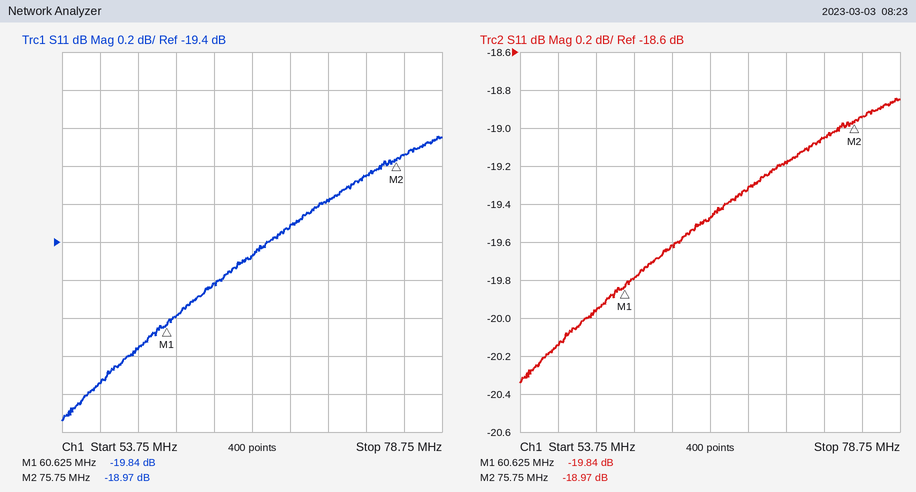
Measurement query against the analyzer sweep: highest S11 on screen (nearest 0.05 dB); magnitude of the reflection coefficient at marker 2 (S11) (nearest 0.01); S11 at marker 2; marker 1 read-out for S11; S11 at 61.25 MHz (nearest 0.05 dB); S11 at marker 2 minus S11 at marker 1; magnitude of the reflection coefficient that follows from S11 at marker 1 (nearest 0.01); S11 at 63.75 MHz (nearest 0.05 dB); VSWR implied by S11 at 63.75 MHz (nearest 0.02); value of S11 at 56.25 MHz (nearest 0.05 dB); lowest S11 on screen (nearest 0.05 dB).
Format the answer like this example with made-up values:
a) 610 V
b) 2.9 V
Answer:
a) -18.85 dB
b) 0.11
c) -18.97 dB
d) -19.84 dB
e) -19.80 dB
f) 0.87 dB
g) 0.10
h) -19.60 dB
i) 1.24
j) -20.15 dB
k) -20.35 dB
